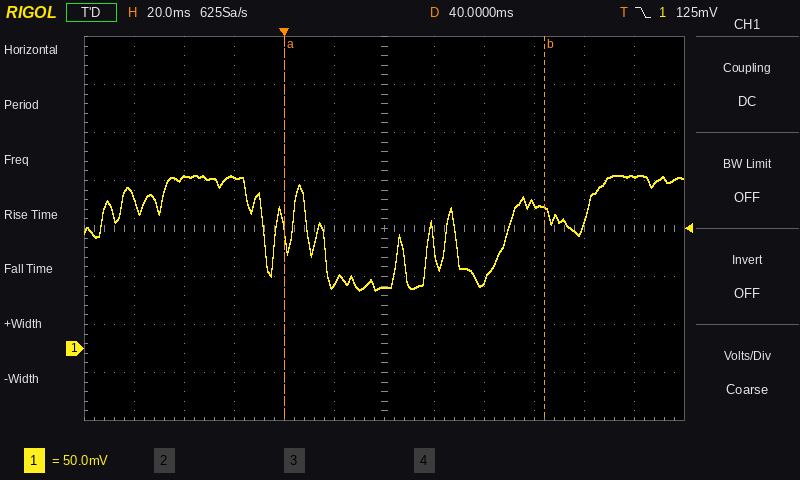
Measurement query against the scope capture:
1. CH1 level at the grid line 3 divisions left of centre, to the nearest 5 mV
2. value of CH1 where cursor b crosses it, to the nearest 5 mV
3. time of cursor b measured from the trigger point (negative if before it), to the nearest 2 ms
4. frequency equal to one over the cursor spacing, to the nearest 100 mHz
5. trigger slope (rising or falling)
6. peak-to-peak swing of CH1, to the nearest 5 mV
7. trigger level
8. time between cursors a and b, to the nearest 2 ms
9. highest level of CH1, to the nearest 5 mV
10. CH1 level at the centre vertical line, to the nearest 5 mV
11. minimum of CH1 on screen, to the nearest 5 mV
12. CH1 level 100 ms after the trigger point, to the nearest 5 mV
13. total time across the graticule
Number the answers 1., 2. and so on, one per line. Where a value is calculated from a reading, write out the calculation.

1. 180 mV
2. 145 mV
3. +104 ms
4. 1 / 104 ms ≈ 9.6 Hz
5. falling
6. 180 mV − (60 mV) = 120 mV
7. 125 mV
8. 104 ms
9. 180 mV
10. 65 mV
11. 60 mV
12. 150 mV
13. 240 ms
